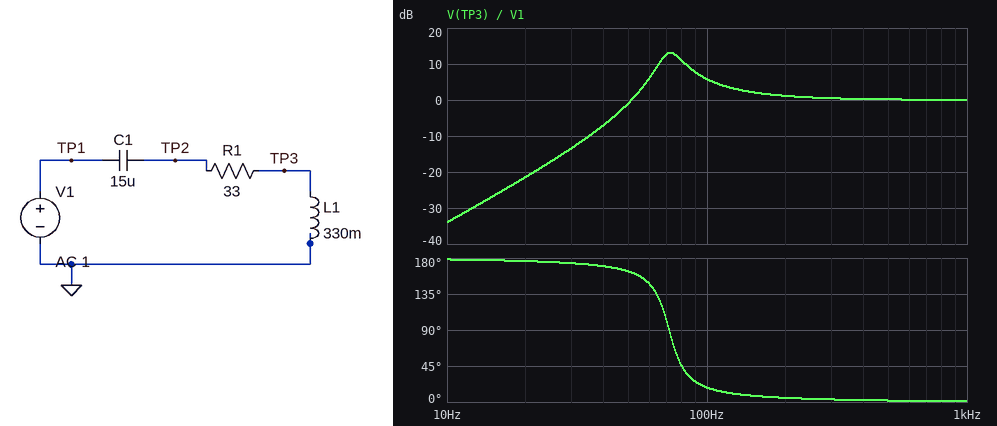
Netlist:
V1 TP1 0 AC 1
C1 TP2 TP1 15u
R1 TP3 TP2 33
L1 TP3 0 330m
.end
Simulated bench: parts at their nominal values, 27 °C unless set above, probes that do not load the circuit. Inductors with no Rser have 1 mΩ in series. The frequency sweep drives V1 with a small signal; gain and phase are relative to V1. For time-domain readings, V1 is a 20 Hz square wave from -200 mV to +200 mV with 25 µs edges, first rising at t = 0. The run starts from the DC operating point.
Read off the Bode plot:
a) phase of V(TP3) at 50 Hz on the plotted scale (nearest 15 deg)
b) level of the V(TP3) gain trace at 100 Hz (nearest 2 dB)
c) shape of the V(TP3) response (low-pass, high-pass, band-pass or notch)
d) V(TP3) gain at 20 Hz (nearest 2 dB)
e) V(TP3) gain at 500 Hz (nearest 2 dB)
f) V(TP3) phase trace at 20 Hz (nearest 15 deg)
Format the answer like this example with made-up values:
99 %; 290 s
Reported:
165 deg; 6 dB; high-pass; -22 dB; 0 dB; 180 deg
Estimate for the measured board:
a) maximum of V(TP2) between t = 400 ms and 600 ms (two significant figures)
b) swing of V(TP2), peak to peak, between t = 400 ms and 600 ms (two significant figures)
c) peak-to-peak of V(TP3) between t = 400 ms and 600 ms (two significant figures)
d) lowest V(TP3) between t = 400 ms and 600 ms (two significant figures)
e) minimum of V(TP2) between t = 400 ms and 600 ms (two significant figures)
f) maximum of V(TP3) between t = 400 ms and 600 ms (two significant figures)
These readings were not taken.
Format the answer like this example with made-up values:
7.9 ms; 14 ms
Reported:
370 mV; 730 mV; 690 mV; -340 mV; -370 mV; 340 mV
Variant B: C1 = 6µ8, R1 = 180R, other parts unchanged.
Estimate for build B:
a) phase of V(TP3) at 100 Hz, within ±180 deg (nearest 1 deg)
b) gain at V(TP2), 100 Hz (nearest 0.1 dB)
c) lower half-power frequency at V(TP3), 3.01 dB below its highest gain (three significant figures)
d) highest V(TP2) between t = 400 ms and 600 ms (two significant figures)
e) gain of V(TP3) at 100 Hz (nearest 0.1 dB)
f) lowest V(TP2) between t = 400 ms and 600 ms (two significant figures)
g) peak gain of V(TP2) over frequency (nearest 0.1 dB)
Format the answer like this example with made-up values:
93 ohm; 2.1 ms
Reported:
98 deg; 3.6 dB; 89.4 Hz; 400 mV; 1.1 dB; -400 mV; 4.3 dB
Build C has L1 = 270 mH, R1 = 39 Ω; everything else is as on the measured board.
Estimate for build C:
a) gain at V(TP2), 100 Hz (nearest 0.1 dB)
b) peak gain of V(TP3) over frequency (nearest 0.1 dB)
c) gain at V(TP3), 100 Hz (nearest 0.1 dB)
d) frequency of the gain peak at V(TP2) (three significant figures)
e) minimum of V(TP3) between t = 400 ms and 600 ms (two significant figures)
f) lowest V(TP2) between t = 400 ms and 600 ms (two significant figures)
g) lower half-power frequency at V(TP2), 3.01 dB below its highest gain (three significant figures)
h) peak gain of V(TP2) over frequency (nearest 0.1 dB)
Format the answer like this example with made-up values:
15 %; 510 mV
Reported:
7.4 dB; 10.8 dB; 7.1 dB; 80.7 Hz; -340 mV; -350 mV; 70.7 Hz; 11.2 dB
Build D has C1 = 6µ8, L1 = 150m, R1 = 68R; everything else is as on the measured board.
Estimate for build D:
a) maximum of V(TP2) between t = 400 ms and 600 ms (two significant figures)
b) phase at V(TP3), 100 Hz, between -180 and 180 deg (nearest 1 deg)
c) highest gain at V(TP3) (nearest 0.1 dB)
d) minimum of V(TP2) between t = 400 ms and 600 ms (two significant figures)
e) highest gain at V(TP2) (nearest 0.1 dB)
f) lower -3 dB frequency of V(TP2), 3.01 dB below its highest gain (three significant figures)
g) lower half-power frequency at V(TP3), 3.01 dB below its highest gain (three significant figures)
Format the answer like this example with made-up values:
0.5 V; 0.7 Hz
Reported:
400 mV; 154 deg; 7.0 dB; -400 mV; 7.8 dB; 134 Hz; 136 Hz
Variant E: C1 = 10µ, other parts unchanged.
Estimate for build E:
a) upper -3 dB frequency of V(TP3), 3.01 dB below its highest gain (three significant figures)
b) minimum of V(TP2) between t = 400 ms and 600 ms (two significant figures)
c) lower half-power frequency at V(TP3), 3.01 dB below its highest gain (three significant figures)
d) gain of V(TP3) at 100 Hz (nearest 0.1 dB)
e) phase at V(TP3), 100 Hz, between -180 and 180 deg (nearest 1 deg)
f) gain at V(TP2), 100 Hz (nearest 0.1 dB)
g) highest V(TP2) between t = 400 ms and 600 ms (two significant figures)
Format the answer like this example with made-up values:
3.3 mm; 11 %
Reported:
97.8 Hz; -340 mV; 81.2 Hz; 11.0 dB; 34 deg; 11.1 dB; 340 mV
